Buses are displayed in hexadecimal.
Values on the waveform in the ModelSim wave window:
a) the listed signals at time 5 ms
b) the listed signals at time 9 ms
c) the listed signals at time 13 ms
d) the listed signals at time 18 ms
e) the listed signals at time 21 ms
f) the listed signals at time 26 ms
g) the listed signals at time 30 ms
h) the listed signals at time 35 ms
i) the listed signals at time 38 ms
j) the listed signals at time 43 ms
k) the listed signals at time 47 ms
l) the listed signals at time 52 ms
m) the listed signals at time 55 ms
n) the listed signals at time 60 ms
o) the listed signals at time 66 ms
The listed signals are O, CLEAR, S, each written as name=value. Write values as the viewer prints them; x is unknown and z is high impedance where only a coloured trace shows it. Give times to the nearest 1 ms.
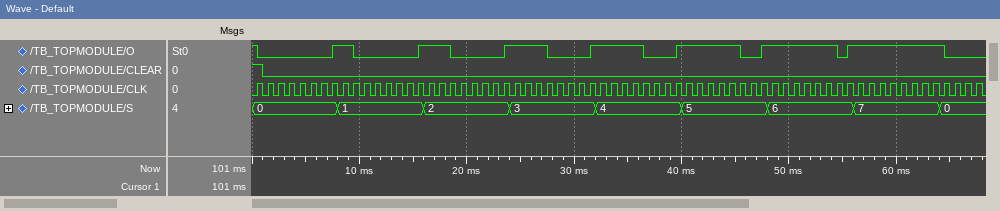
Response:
O=0, CLEAR=0, S=0
O=1, CLEAR=0, S=1
O=0, CLEAR=0, S=1
O=1, CLEAR=0, S=2
O=0, CLEAR=0, S=2
O=1, CLEAR=0, S=3
O=0, CLEAR=0, S=3
O=1, CLEAR=0, S=4
O=0, CLEAR=0, S=4
O=1, CLEAR=0, S=5
O=0, CLEAR=0, S=5
O=1, CLEAR=0, S=6
O=0, CLEAR=0, S=6
O=1, CLEAR=0, S=7
O=0, CLEAR=0, S=0
